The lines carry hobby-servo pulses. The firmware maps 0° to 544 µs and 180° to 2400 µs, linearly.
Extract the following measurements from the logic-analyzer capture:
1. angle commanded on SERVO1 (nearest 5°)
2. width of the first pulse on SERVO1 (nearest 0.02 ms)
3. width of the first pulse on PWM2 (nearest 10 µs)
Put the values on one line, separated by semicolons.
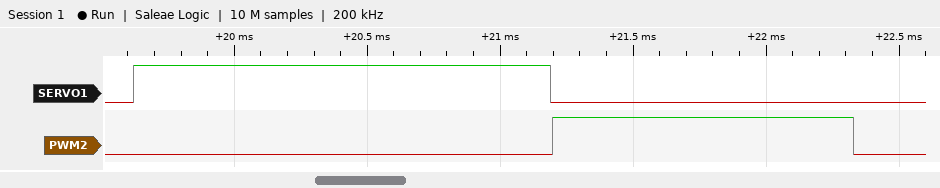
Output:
100°; 1.56 ms; 1130 µs
